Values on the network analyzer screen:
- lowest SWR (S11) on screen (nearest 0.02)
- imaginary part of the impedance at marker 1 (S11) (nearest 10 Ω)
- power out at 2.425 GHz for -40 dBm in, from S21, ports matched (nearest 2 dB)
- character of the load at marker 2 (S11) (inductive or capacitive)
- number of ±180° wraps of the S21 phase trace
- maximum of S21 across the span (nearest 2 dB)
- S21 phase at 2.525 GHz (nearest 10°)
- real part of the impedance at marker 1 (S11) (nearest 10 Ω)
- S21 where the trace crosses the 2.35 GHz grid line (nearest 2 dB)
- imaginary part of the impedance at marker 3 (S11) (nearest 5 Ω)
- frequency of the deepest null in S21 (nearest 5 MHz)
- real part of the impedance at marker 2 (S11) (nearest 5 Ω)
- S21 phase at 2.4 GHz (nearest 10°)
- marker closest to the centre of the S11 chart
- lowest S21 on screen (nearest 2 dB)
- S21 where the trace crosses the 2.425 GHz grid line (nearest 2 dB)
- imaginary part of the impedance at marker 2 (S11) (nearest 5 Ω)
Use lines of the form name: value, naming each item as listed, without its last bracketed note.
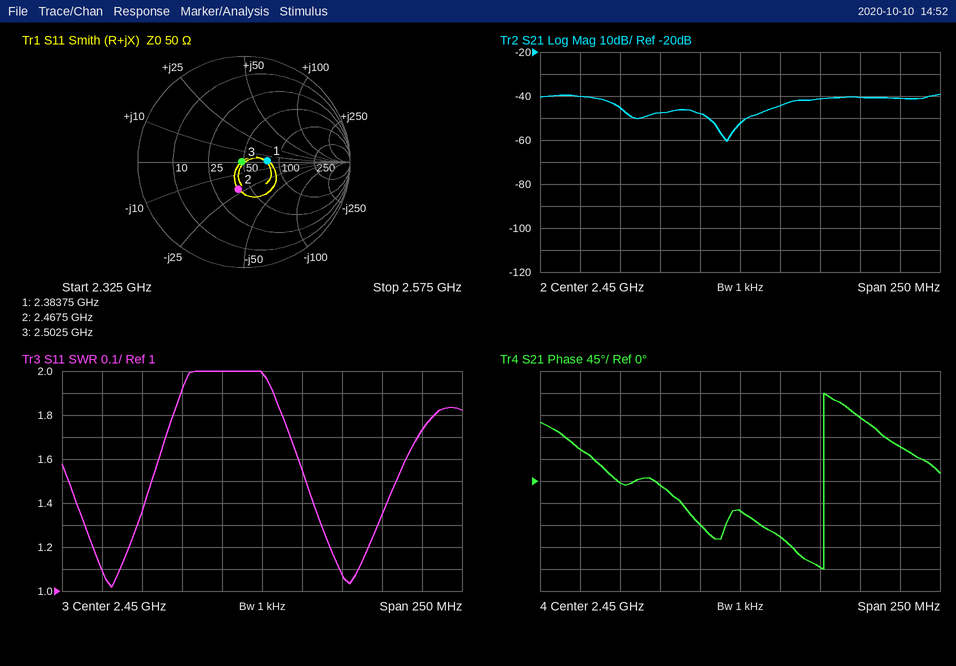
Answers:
lowest SWR (S11) on screen: 1.02
imaginary part of the impedance at marker 1 (S11): 0 Ω
power out at 2.425 GHz for -40 dBm in, from S21, ports matched: -88 dBm
character of the load at marker 2 (S11): capacitive
number of ±180° wraps of the S21 phase trace: 1
maximum of S21 across the span: -40 dB
S21 phase at 2.525 GHz: 130°
real part of the impedance at marker 1 (S11): 80 Ω
S21 where the trace crosses the 2.35 GHz grid line: -40 dB
imaginary part of the impedance at marker 3 (S11): 0 Ω
frequency of the deepest null in S21: 2.440 GHz
real part of the impedance at marker 2 (S11): 40 Ω
S21 phase at 2.4 GHz: -10°
marker closest to the centre of the S11 chart: marker 3
lowest S21 on screen: -60 dB
S21 where the trace crosses the 2.425 GHz grid line: -48 dB
imaginary part of the impedance at marker 2 (S11): -20 Ω
